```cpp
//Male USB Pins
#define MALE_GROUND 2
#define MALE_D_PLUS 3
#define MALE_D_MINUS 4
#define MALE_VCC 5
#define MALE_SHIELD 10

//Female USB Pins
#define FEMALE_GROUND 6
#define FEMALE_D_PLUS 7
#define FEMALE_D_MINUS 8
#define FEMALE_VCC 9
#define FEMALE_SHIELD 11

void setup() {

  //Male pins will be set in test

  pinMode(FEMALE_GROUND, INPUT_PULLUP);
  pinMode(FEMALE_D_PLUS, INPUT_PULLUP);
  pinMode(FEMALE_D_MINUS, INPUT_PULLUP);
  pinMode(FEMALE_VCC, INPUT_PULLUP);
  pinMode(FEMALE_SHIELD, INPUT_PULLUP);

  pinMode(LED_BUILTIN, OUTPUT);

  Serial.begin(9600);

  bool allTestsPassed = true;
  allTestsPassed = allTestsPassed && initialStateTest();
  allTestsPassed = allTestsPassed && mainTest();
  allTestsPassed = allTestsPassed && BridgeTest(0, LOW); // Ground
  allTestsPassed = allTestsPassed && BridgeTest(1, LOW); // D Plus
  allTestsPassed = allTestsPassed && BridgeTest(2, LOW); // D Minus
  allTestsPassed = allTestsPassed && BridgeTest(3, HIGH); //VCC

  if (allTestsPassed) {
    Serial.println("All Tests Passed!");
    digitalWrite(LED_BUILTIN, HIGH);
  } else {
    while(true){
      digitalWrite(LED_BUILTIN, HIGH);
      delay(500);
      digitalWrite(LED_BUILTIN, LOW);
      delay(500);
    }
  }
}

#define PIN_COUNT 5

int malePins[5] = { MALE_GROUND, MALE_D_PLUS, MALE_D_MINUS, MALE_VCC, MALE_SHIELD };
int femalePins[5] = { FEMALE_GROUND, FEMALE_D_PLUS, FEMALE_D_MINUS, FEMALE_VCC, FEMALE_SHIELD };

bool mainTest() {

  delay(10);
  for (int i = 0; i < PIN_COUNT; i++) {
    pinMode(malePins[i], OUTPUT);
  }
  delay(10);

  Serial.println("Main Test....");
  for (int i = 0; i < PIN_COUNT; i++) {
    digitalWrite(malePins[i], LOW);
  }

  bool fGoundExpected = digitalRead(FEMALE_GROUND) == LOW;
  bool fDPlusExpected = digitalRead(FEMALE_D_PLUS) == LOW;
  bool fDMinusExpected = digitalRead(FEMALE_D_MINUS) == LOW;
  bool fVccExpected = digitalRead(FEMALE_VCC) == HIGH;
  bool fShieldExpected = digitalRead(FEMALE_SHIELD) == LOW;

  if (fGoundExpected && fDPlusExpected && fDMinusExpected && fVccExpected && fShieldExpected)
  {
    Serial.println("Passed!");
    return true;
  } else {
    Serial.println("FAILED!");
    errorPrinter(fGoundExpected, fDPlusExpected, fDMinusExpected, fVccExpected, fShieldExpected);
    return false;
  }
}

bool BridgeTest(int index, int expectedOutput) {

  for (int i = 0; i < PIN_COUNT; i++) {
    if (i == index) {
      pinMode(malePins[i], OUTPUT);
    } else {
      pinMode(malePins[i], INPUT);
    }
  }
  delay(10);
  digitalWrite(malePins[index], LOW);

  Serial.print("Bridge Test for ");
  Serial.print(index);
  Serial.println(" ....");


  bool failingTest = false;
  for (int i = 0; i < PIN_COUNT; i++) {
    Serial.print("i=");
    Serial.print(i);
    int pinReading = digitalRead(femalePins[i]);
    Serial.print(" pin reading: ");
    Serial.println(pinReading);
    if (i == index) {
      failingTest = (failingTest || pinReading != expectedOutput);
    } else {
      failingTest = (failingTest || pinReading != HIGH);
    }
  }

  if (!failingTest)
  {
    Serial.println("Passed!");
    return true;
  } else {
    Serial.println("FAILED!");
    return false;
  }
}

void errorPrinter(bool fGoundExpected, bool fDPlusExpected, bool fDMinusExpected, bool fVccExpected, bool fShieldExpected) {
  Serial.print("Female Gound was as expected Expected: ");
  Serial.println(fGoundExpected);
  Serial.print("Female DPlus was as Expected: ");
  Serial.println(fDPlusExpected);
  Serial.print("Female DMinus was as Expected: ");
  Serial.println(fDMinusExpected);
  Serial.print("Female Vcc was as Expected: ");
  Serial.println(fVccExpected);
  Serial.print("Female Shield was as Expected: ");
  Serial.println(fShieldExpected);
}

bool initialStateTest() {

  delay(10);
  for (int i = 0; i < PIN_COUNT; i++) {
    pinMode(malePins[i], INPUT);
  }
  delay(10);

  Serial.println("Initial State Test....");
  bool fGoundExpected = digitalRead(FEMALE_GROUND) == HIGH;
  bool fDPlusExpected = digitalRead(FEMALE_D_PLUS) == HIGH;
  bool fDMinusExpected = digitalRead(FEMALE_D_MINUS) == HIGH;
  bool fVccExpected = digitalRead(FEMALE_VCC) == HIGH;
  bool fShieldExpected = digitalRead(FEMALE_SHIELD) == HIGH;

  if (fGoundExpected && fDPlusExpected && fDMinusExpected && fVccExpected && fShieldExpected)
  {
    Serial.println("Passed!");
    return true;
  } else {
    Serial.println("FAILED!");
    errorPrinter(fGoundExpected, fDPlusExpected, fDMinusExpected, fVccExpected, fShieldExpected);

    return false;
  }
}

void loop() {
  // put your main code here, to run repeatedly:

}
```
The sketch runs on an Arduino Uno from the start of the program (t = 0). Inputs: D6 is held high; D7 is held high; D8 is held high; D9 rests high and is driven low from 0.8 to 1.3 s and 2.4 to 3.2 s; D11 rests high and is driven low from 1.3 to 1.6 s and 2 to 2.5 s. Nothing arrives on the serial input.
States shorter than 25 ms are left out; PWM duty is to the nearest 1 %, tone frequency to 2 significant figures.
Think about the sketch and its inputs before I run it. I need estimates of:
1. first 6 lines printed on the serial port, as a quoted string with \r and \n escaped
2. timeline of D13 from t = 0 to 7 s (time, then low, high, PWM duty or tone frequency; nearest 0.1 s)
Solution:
"Initial State Test....\r\nPassed!\r\nMain Test....\r\nFAILED!\r\nFemale Gound was as expected Expected: 0\r\nFemale DPlus was as Expected: 0\r\n"
0 s low; 0.2 s high; 0.7 s low; 1.2 s high; 1.7 s low; 2.2 s high; 2.7 s low; 3.2 s high; 3.7 s low; 4.2 s high; 4.7 s low; 5.2 s high; 5.7 s low; 6.2 s high; 6.7 s low
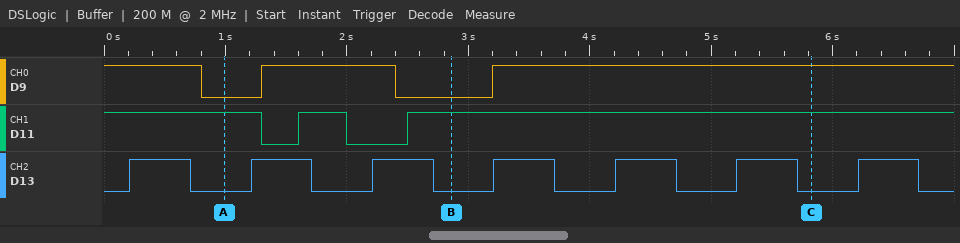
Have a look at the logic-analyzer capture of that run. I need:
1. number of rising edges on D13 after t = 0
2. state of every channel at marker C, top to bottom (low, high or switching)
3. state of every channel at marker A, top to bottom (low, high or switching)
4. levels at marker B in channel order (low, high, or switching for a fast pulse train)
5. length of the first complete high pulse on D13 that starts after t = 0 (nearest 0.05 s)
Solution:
7
D9 high, D11 high, D13 low
D9 low, D11 high, D13 low
D9 low, D11 high, D13 low
0.50 s
